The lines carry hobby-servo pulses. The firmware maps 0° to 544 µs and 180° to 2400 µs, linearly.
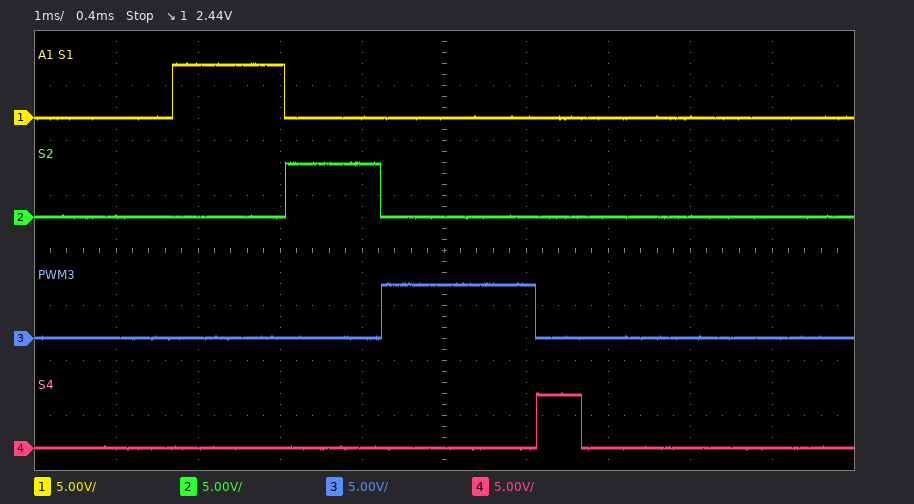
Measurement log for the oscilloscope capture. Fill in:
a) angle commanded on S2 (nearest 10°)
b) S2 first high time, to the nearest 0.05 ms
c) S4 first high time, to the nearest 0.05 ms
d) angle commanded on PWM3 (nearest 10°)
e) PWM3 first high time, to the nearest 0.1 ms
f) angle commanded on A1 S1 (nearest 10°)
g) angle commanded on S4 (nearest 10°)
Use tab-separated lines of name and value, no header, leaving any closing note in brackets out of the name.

angle commanded on S2	60°
S2 first high time, to the nearest 0.05 ms	1.15 ms
S4 first high time, to the nearest 0.05 ms	0.55 ms
angle commanded on PWM3	130°
PWM3 first high time, to the nearest 0.1 ms	1.9 ms
angle commanded on A1 S1	80°
angle commanded on S4	0°
